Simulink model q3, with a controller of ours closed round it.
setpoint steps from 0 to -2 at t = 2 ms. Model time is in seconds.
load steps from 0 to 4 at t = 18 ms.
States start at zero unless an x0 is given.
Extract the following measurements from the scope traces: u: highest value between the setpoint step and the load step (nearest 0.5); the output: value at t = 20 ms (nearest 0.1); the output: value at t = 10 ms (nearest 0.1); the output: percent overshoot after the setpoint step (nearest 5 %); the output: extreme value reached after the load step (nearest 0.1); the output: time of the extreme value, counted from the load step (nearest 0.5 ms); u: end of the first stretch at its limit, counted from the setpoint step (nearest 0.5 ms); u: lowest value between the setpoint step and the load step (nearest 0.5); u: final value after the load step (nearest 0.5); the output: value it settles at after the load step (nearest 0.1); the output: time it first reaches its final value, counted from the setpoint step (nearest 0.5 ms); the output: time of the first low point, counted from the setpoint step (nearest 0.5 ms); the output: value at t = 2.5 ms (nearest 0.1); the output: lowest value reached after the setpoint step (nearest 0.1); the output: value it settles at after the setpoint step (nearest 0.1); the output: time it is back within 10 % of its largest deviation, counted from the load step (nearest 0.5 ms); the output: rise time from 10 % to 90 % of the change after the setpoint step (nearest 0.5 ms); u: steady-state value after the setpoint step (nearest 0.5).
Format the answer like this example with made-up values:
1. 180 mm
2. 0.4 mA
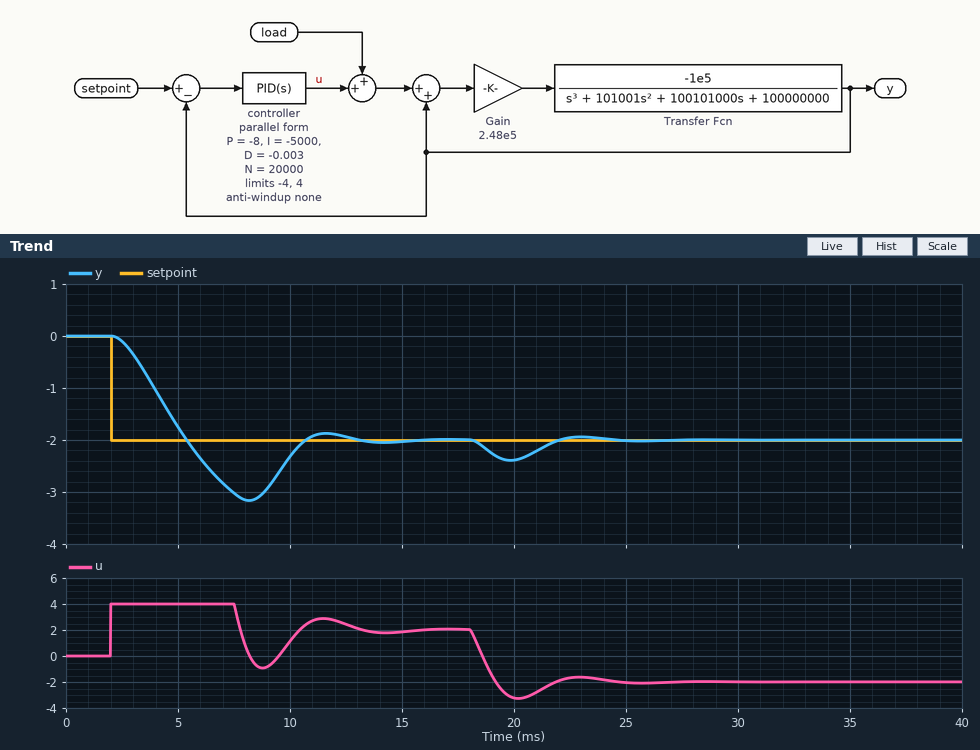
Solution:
1. 4.0
2. -2.4
3. -2.3
4. 60 %
5. -2.4
6. 2.0 ms
7. 5.5 ms
8. -1.0
9. -2.0
10. -2.0
11. 3.5 ms
12. 6.0 ms
13. -0.1
14. -3.2
15. -2.0
16. 5.5 ms
17. 2.5 ms
18. 2.0
